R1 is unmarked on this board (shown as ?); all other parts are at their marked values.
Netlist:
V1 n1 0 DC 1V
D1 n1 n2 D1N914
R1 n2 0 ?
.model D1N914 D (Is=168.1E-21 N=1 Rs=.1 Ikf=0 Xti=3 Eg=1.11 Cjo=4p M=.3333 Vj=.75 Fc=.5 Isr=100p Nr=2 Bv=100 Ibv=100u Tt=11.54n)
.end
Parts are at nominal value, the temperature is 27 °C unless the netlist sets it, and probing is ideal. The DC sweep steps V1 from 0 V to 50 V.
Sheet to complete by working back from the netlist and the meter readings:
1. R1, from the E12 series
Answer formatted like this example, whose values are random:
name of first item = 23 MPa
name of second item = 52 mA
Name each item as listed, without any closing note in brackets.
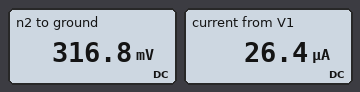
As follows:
R1, from the E12 series = 12 kΩ
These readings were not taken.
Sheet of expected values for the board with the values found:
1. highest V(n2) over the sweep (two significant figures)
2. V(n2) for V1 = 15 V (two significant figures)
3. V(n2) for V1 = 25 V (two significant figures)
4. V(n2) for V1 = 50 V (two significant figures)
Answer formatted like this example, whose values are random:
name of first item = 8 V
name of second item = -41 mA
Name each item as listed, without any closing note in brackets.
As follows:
highest V(n2) over the sweep = 49 V
V(n2) for V1 = 15 V = 14 V
V(n2) for V1 = 25 V = 24 V
V(n2) for V1 = 50 V = 49 V
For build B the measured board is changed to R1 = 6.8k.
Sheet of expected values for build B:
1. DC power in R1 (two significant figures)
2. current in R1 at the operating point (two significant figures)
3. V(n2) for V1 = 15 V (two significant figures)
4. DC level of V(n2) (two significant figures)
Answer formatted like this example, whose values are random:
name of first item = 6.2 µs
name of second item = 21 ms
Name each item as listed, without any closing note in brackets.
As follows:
DC power in R1 = 12 µW
current in R1 at the operating point = 42 µA
V(n2) for V1 = 15 V = 14 V
DC level of V(n2) = 290 mV
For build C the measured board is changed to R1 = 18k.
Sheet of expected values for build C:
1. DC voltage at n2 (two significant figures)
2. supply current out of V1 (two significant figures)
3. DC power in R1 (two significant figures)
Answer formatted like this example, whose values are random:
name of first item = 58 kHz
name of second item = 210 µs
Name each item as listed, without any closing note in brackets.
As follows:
DC voltage at n2 = 340 mV
supply current out of V1 = 19 µA
DC power in R1 = 6.3 µW
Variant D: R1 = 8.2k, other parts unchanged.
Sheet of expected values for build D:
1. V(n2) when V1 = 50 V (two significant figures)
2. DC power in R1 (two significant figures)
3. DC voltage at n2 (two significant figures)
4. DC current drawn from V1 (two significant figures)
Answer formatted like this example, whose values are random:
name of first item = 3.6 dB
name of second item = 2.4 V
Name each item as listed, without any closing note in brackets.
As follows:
V(n2) when V1 = 50 V = 49 V
DC power in R1 = 11 µW
DC voltage at n2 = 300 mV
DC current drawn from V1 = 36 µA
